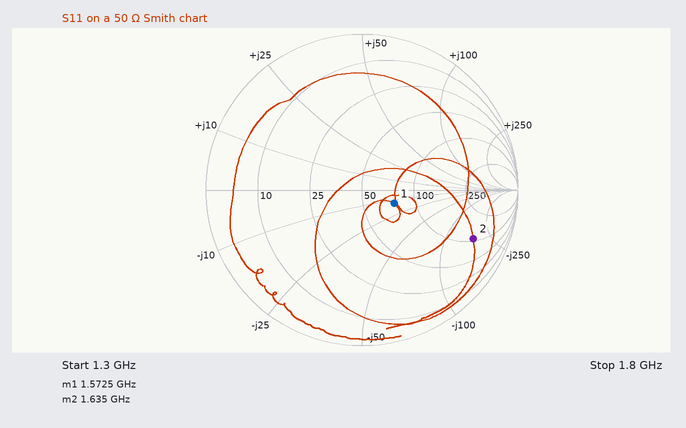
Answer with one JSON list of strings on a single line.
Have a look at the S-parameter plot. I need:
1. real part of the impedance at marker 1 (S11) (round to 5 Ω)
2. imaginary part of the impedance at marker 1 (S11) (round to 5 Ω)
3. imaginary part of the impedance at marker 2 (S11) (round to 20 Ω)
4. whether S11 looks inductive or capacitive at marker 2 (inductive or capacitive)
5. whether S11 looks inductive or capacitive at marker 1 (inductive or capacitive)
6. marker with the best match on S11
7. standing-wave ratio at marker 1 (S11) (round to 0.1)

["75 Ω", "-15 Ω", "-180 Ω", "capacitive", "capacitive", "marker 1", "1.6"]
